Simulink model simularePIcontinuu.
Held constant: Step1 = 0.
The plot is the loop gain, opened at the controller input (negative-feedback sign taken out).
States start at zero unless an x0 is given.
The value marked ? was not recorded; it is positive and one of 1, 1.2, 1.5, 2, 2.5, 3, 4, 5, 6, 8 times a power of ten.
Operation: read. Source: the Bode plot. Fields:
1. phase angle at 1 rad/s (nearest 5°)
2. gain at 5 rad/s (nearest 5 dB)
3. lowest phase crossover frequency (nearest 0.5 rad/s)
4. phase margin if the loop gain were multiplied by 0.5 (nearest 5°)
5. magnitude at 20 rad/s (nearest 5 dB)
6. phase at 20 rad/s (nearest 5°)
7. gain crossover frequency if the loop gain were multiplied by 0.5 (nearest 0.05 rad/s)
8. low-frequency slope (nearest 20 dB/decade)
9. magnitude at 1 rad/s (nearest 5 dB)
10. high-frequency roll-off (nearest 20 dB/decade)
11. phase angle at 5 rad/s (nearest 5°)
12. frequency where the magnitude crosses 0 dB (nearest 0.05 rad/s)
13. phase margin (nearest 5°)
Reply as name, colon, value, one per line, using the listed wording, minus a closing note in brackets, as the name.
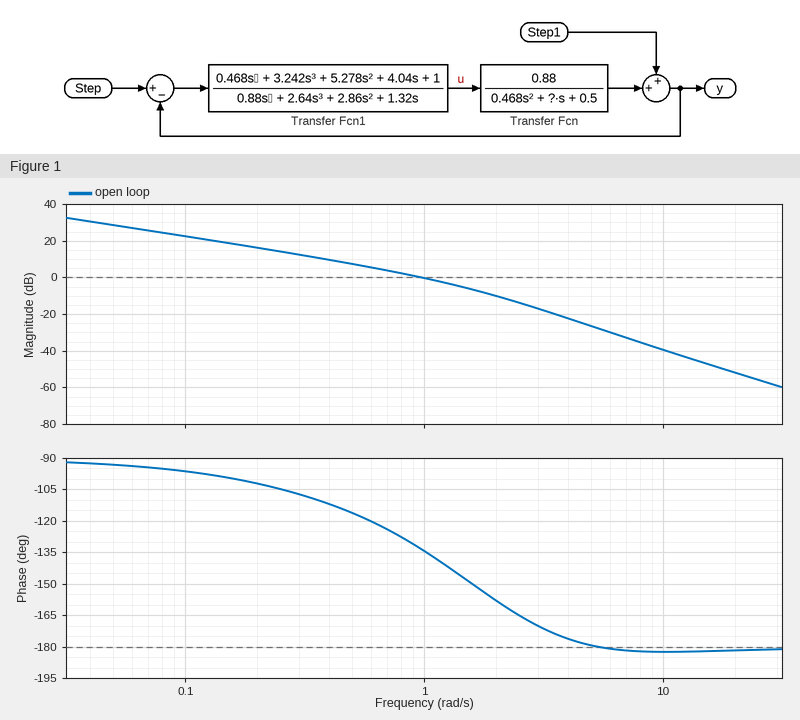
phase angle at 1 rad/s: -135°
gain at 5 rad/s: -25 dB
lowest phase crossover frequency: 5.5 rad/s
phase margin if the loop gain were multiplied by 0.5: 60°
magnitude at 20 rad/s: -50 dB
phase at 20 rad/s: -180°
gain crossover frequency if the loop gain were multiplied by 0.5: 0.55 rad/s
low-frequency slope: -20 dB/decade
magnitude at 1 rad/s: 0 dB
high-frequency roll-off: -40 dB/decade
phase angle at 5 rad/s: -180°
frequency where the magnitude crosses 0 dB: 0.95 rad/s
phase margin: 45°
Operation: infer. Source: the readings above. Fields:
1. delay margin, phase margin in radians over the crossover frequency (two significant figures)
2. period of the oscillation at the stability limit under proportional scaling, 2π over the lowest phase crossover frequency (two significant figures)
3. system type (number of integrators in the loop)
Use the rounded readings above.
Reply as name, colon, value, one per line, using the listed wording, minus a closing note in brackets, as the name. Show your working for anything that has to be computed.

delay margin, phase margin in radians over the crossover frequency: 45 × π / 180 / 0.95 = 0.83 s
period of the oscillation at the stability limit under proportional scaling, 2π over the lowest phase crossover frequency: 2π / 5.5 = 1.1 s
system type: 1
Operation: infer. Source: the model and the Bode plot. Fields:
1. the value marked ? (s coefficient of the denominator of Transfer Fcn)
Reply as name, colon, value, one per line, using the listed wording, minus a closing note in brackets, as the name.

the value marked ?: 1.5
